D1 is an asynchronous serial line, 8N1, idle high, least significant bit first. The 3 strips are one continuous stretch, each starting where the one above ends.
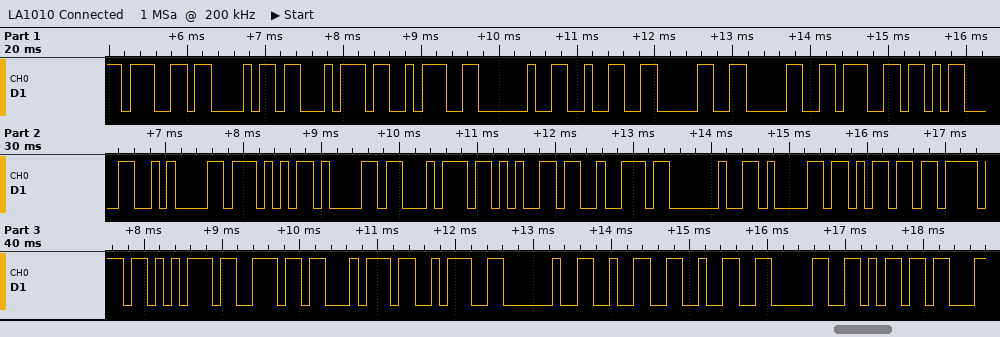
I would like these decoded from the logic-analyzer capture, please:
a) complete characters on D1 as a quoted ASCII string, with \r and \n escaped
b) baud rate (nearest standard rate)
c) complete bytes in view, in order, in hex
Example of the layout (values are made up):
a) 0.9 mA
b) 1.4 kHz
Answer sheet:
a) "ght: 200g\r\nWater amount: 220m"
b) 9600 baud
c) 67 68 74 3A 20 32 30 30 67 0D 0A 57 61 74 65 72 20 61 6D 6F 75 6E 74 3A 20 32 32 30 6D
